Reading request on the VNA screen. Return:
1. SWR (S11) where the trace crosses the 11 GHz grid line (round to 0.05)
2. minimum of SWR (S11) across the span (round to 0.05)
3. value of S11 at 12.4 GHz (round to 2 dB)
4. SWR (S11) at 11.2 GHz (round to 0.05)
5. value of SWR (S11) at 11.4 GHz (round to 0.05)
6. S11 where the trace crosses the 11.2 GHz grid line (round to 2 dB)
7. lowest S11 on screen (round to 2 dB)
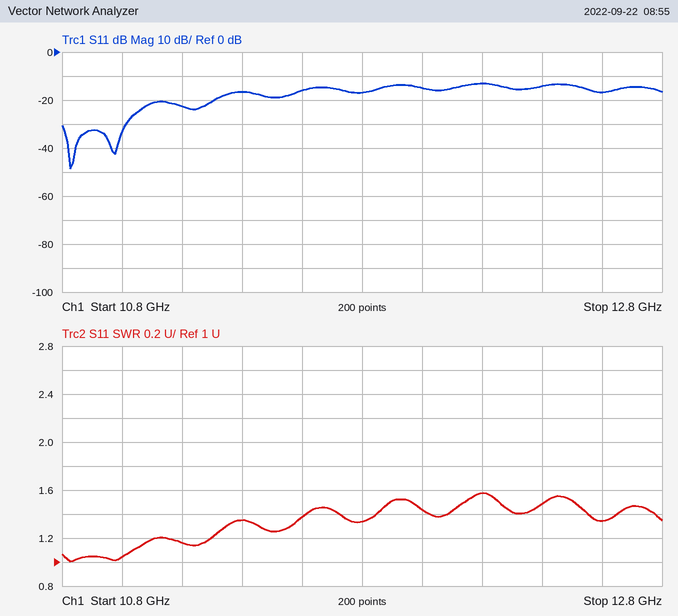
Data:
1.05
1.00
-14 dB
1.15
1.35
-22 dB
-48 dB
